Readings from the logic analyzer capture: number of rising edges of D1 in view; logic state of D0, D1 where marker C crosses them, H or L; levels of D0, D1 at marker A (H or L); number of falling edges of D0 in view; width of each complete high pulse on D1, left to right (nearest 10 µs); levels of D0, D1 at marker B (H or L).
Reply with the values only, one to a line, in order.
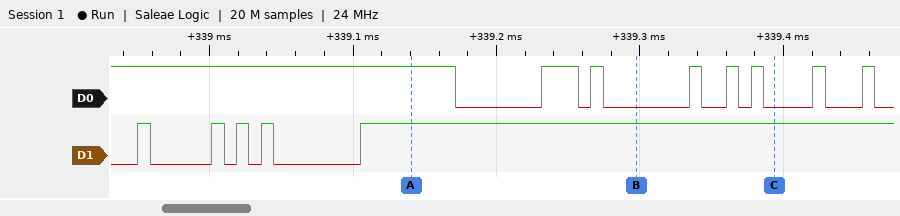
5
D0=L, D1=H
D0=H, D1=H
8
10 µs, 10 µs, 10 µs, 10 µs
D0=L, D1=H
